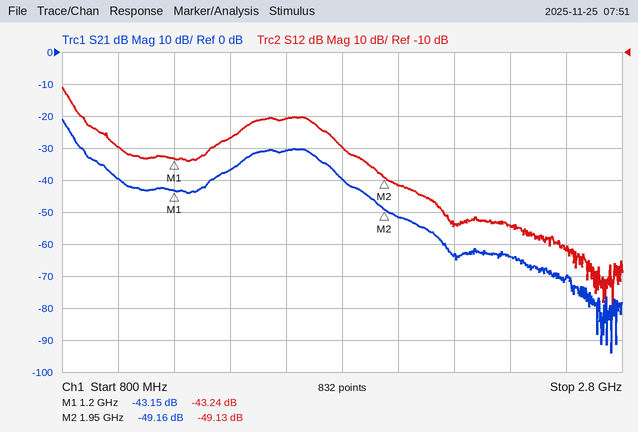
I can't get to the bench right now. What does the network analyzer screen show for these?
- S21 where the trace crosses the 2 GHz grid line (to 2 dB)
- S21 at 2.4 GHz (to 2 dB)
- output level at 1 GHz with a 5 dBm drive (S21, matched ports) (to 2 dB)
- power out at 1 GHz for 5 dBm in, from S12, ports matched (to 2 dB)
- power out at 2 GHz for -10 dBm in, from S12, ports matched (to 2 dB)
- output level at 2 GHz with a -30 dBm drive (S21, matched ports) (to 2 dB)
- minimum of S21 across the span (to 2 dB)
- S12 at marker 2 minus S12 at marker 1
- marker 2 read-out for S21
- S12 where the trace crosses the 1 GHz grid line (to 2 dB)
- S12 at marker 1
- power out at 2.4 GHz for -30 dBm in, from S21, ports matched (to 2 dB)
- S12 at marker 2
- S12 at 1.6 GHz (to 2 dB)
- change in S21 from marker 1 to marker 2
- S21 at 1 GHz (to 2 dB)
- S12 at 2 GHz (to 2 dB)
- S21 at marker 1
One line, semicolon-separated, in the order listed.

-52 dB; -64 dB; -34 dBm; -34 dBm; -62 dBm; -82 dBm; -94 dB; -5.89 dB; -49.16 dB; -40 dB; -43.24 dB; -94 dBm; -49.13 dB; -30 dB; -6.01 dB; -40 dB; -52 dB; -43.15 dB
